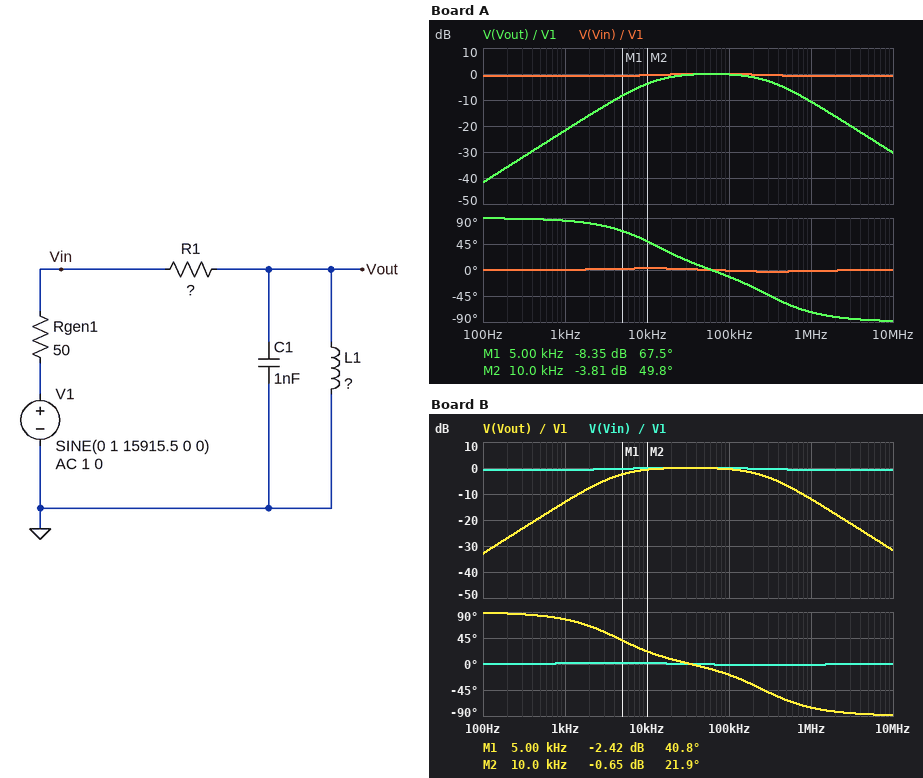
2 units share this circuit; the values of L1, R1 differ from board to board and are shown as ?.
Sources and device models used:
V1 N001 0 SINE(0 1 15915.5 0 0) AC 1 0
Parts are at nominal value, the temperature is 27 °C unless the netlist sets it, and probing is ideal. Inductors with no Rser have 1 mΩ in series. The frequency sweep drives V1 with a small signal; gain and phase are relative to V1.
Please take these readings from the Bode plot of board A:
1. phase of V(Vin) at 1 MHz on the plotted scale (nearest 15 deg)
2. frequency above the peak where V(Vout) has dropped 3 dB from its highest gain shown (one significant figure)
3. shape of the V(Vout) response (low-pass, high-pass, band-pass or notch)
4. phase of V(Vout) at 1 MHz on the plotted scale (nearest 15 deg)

0 deg
300 kHz
band-pass
-75 deg
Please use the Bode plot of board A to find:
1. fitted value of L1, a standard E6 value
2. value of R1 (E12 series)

6.8 mH
470 Ω
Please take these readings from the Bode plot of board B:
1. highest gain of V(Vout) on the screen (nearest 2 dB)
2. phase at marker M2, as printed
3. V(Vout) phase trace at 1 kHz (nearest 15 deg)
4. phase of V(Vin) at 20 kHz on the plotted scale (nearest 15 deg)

0 dB
21.9 deg
75 deg
0 deg
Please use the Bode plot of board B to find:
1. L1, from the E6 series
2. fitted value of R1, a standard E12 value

22 mH
560 Ω
